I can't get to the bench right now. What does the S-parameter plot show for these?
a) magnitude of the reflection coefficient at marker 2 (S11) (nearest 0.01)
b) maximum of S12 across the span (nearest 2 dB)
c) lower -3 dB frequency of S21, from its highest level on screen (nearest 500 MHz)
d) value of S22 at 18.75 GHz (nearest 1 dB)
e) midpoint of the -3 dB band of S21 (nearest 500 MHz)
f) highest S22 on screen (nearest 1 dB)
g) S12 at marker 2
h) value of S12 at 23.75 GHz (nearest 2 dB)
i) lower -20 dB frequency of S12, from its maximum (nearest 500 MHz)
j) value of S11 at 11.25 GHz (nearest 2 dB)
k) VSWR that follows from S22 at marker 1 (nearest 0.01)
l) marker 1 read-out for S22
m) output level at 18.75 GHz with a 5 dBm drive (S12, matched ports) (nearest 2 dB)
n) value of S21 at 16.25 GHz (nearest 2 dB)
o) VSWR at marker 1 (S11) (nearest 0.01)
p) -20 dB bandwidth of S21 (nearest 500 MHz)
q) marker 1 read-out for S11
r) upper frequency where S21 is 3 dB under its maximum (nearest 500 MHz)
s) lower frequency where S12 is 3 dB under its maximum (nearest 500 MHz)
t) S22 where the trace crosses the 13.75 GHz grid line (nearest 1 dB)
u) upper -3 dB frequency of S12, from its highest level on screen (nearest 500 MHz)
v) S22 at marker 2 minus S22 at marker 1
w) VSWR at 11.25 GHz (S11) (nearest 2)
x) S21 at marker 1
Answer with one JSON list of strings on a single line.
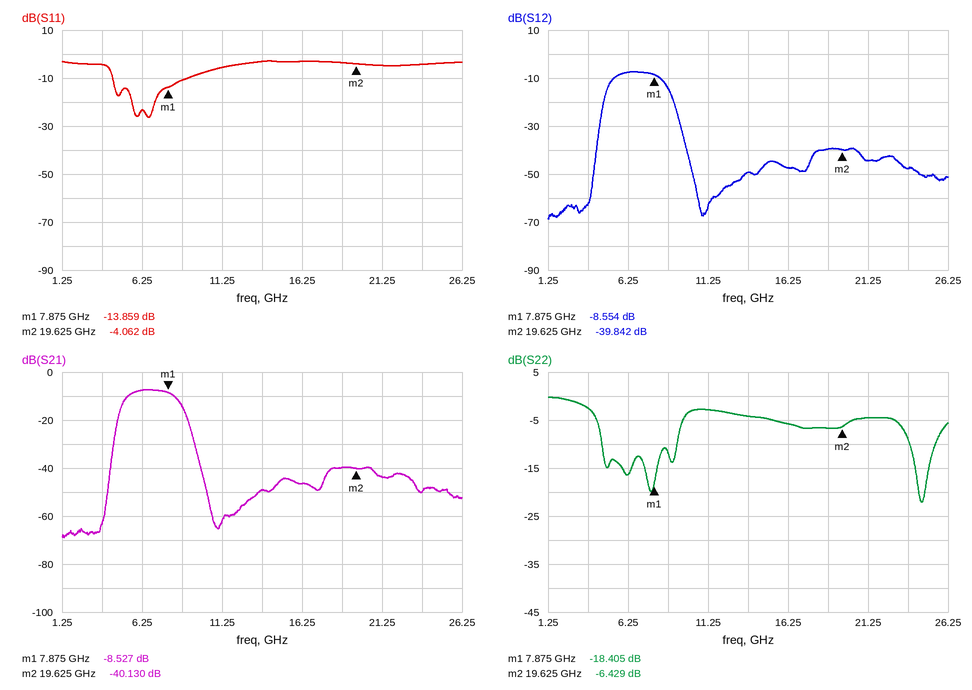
["0.63", "-8 dB", "5.5 GHz", "-7 dB", "7.0 GHz", "0 dB", "-39.842 dB", "-48 dB", "4.5 GHz", "-6 dB", "1.27", "-18.405 dB", "-34 dBm", "-46 dB", "1.51", "5.0 GHz", "-13.859 dB", "8.5 GHz", "5.5 GHz", "-4 dB", "8.5 GHz", "11.976 dB", "4", "-8.527 dB"]
